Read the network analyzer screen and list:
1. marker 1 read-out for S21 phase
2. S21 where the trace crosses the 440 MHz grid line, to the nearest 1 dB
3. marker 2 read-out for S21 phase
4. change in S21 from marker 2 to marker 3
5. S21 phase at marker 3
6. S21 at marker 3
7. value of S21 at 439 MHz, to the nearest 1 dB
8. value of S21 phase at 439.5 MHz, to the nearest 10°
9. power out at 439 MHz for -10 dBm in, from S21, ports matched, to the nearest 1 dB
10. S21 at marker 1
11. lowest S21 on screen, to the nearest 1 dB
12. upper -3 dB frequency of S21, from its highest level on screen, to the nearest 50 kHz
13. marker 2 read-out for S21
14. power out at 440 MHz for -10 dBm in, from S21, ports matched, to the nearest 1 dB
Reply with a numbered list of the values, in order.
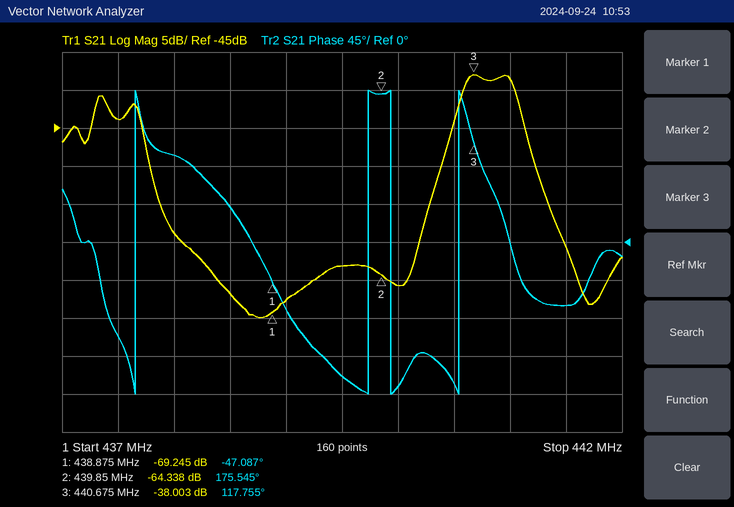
1. -47.087°
2. -66 dB
3. 175.545°
4. 26.335 dB
5. 117.755°
6. -38.003 dB
7. -68 dB
8. -160°
9. -78 dBm
10. -69.245 dB
11. -70 dB
12. 441.05 MHz
13. -64.338 dB
14. -76 dBm
